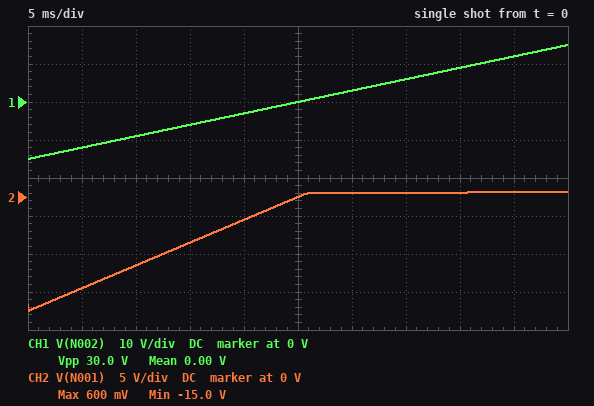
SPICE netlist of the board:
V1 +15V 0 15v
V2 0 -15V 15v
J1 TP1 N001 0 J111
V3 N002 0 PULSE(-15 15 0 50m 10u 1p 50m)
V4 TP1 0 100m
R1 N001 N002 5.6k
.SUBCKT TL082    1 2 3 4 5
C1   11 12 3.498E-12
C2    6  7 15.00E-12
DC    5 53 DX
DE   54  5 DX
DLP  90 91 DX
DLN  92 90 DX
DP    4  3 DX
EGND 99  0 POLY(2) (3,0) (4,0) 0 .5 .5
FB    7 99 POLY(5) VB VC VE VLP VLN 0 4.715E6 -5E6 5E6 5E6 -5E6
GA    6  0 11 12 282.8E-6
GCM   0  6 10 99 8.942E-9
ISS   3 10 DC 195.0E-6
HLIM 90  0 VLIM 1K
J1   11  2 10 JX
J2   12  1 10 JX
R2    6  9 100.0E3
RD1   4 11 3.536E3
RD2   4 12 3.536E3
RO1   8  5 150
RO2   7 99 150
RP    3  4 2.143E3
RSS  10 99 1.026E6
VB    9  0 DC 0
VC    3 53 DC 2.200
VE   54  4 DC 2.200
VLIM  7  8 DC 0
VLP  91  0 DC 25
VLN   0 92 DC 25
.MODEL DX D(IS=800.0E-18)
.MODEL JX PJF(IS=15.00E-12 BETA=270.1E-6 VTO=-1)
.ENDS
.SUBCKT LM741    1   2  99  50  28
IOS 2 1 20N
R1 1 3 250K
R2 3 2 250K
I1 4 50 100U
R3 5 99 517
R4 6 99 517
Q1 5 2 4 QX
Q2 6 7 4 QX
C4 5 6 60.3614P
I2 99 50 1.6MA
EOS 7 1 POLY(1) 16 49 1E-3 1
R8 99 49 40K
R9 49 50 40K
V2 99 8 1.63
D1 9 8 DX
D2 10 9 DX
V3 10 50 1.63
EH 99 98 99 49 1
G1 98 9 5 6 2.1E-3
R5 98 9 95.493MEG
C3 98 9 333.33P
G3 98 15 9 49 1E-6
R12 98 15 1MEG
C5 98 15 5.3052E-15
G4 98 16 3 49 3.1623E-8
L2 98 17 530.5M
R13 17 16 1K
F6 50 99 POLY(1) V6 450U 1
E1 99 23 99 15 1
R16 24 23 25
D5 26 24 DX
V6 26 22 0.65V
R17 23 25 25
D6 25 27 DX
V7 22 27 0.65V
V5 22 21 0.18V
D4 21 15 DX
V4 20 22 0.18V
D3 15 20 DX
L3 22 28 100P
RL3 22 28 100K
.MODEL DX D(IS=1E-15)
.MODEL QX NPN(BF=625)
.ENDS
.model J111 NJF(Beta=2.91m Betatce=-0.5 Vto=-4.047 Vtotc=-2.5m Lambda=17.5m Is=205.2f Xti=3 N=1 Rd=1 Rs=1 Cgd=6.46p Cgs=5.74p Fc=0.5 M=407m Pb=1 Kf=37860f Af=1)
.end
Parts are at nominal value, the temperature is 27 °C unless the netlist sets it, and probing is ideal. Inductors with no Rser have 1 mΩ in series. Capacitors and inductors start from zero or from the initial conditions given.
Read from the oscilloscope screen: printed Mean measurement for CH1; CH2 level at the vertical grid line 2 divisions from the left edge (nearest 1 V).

0.00 V
-9 V
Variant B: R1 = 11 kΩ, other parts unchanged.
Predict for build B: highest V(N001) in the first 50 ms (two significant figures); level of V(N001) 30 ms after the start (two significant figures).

590 mV
540 mV
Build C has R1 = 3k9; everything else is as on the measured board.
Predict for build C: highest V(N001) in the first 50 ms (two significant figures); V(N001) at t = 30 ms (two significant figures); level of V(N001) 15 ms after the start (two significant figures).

620 mV
570 mV
-6.0 V
